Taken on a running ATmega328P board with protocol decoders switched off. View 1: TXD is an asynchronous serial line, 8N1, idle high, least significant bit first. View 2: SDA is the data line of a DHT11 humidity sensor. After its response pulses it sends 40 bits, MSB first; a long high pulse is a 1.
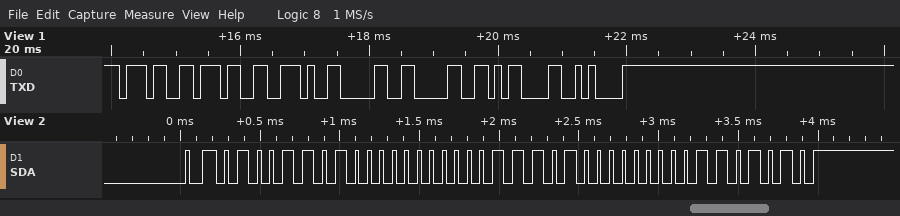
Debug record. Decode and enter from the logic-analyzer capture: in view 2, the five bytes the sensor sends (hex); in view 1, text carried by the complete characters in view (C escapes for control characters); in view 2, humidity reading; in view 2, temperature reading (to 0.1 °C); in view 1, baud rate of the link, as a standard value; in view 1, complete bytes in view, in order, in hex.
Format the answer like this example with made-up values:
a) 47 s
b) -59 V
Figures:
a) 4D 00 1D 00 6A
b) "77.00\r\n"
c) 77 %
d) 29.0 °C
e) 9600 baud
f) 37 37 2E 30 30 0D 0A
